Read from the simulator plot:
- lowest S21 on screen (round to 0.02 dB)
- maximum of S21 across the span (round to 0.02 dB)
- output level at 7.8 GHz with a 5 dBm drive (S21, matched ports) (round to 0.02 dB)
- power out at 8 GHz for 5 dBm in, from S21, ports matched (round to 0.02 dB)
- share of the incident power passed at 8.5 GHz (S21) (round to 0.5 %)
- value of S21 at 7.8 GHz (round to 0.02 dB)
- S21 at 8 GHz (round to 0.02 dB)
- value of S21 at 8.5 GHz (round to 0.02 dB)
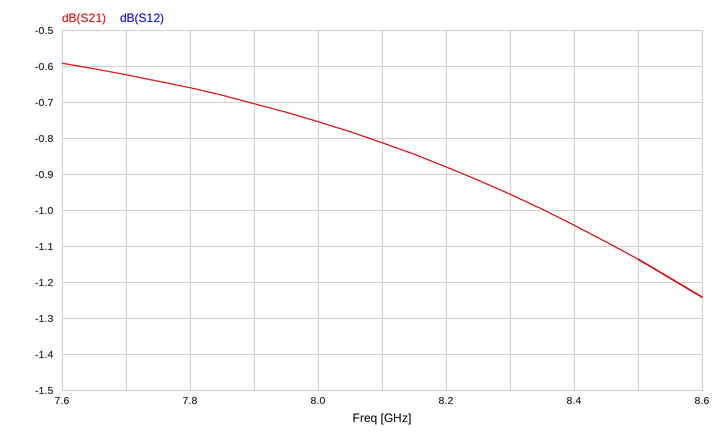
-1.24 dB
-0.60 dB
4.34 dBm
4.24 dBm
77.0 %
-0.66 dB
-0.76 dB
-1.14 dB
